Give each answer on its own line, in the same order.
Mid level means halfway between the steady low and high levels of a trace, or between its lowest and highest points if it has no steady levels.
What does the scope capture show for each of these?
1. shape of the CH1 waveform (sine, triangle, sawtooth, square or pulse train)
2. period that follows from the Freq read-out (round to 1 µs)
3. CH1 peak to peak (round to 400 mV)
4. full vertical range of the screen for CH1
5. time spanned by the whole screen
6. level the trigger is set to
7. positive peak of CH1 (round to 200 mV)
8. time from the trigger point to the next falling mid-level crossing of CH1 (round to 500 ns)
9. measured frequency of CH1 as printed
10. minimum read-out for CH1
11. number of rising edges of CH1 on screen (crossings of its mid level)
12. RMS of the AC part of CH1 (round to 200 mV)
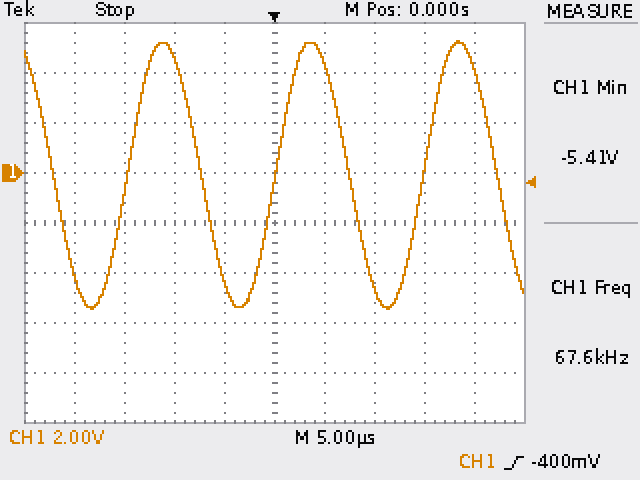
sine
15 µs
10.8 V
16 V
50 µs
-400 mV
5.2 V
7.5 µs
67.6 kHz
-5.41 V
3
3.8 V
